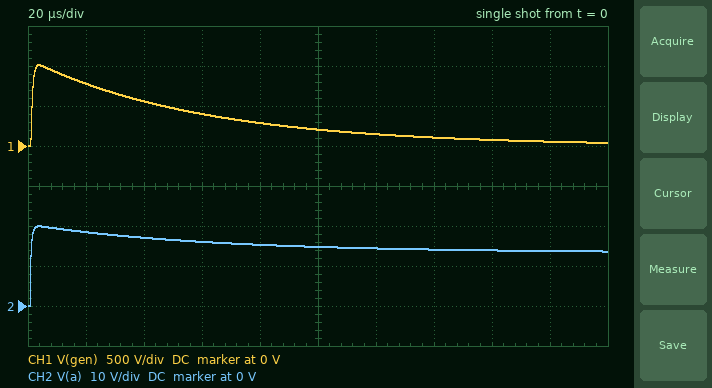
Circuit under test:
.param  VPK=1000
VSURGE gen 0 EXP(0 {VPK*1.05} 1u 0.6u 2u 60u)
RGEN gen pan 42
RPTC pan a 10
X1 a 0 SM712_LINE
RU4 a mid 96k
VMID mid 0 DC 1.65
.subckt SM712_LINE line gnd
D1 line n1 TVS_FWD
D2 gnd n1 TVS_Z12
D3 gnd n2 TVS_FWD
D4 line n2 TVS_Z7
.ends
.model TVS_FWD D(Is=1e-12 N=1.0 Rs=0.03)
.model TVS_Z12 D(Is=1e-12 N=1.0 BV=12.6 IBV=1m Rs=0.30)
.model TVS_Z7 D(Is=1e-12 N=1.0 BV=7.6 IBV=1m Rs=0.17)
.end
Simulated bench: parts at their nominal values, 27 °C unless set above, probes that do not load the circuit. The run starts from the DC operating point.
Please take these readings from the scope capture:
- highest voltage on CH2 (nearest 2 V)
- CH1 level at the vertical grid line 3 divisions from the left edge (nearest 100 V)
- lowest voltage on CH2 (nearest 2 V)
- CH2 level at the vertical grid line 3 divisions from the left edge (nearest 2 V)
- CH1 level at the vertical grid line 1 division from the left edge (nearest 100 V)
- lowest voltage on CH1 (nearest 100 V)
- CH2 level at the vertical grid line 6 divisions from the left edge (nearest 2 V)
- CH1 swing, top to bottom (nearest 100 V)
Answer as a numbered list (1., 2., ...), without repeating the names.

1. 20 V
2. 400 V
3. 0 V
4. 16 V
5. 800 V
6. 0 V
7. 14 V
8. 1.0 kV
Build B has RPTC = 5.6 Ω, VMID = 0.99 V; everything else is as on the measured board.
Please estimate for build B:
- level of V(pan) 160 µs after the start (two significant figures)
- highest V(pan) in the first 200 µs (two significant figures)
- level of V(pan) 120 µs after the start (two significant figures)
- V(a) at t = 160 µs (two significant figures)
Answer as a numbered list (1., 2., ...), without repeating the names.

1. 21 V
2. 140 V
3. 30 V
4. 14 V
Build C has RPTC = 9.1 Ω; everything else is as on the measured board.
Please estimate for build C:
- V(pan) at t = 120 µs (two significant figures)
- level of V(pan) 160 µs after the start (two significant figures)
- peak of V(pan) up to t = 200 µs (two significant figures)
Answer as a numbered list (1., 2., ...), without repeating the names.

1. 38 V
2. 25 V
3. 200 V
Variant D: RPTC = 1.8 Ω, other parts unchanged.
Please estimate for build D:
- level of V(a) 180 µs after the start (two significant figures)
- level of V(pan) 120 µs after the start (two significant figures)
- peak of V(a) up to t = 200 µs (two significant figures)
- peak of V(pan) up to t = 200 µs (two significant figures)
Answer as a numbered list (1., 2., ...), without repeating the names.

1. 14 V
2. 20 V
3. 21 V
4. 62 V
